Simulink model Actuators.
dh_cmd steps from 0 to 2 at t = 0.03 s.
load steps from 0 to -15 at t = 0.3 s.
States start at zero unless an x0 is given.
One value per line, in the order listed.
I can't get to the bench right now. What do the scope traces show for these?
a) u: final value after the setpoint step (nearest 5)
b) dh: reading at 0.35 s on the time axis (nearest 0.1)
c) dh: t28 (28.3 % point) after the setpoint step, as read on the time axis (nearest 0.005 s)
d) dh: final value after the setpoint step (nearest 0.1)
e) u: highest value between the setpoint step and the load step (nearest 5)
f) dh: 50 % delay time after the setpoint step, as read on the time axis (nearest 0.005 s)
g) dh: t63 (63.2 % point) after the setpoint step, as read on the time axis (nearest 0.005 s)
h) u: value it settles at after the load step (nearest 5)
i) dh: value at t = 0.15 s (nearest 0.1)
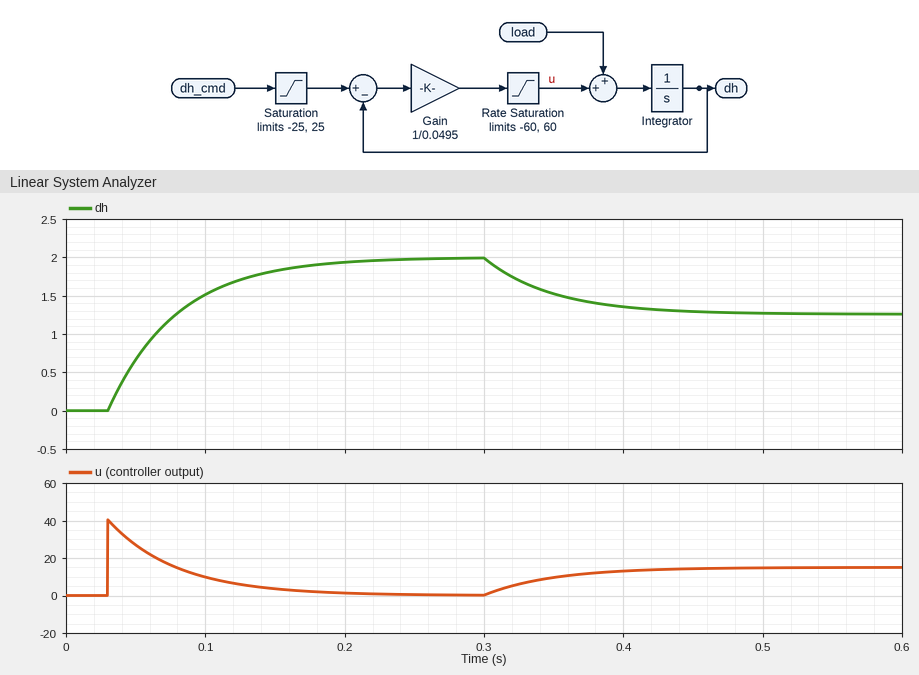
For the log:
0
1.5
0.045 s
2.0
40
0.065 s
0.080 s
15
1.8
